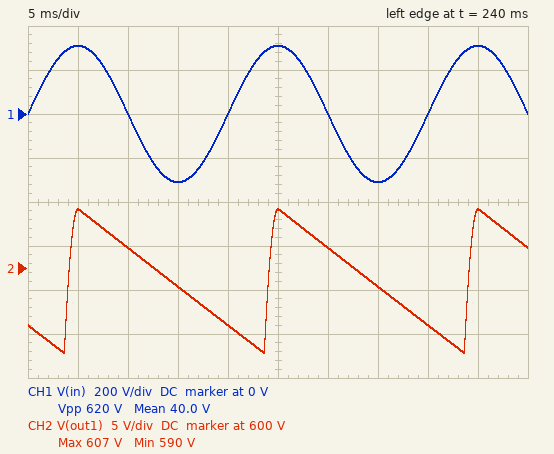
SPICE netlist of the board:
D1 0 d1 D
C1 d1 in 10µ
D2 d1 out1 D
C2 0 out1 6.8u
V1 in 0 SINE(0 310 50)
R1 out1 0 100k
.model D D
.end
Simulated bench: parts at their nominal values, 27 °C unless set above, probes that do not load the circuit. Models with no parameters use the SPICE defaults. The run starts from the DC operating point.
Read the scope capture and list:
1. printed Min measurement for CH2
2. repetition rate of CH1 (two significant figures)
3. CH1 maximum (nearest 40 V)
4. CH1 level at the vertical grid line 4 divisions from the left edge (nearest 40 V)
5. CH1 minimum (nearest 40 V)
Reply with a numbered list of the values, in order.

1. 590 V
2. 50 Hz
3. 320 V
4. 0 V
5. -320 V
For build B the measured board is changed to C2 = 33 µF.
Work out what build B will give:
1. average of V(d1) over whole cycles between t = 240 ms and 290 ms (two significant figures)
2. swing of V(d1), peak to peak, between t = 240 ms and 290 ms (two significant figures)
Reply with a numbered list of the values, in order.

1. 290 V
2. 600 V
